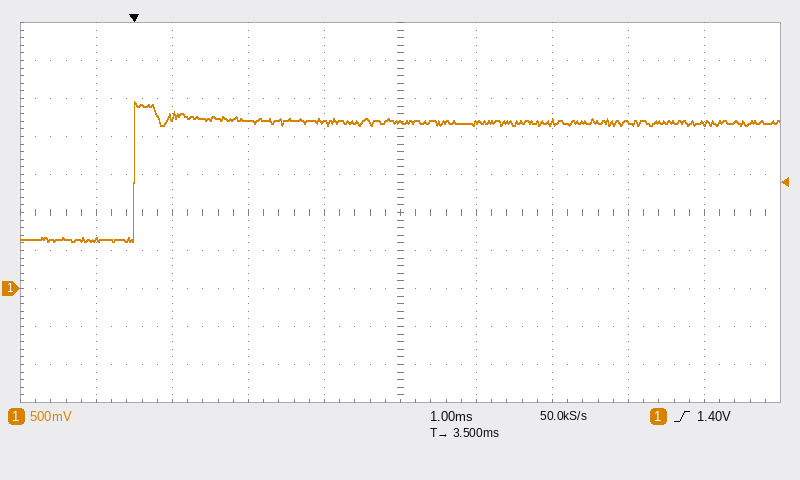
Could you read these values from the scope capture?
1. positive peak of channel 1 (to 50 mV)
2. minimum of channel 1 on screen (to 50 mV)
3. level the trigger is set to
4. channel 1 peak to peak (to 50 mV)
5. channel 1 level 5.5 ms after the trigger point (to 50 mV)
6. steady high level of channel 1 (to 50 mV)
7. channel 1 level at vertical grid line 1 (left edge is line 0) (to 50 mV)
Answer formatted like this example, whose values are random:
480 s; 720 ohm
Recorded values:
2.45 V; 600 mV; 1.40 V; 1.85 V; 2.20 V; 2.20 V; 650 mV
